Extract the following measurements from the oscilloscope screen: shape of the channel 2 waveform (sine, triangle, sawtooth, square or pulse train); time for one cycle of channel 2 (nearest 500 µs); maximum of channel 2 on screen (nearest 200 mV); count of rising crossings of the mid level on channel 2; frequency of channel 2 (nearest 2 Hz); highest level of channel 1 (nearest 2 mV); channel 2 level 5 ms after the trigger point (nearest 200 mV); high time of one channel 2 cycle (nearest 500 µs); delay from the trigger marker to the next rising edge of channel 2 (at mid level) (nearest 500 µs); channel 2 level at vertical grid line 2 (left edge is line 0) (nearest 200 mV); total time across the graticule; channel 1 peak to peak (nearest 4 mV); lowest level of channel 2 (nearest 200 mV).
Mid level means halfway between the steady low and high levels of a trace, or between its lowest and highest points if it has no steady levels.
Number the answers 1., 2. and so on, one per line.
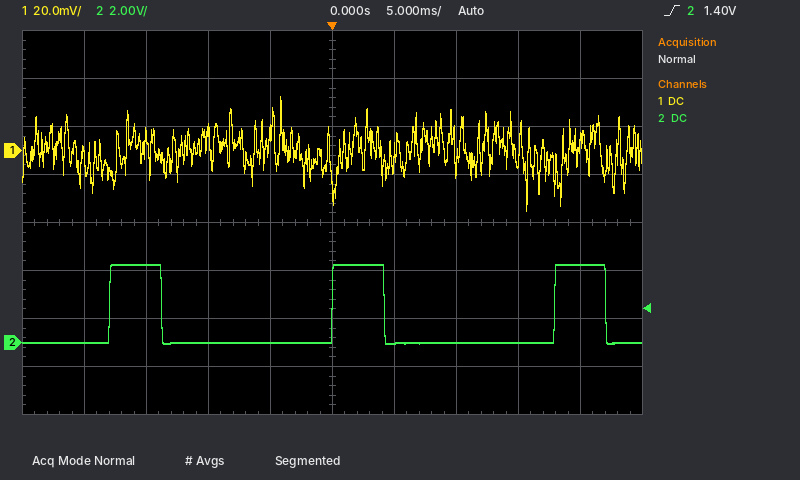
1. pulse train
2. 18.0 ms
3. 3.2 V
4. 3
5. 56 Hz
6. 22 mV
7. 0.0 V
8. 4.0 ms
9. 18.0 ms
10. 3.2 V
11. 50 ms
12. 48 mV
13. 0.0 V
